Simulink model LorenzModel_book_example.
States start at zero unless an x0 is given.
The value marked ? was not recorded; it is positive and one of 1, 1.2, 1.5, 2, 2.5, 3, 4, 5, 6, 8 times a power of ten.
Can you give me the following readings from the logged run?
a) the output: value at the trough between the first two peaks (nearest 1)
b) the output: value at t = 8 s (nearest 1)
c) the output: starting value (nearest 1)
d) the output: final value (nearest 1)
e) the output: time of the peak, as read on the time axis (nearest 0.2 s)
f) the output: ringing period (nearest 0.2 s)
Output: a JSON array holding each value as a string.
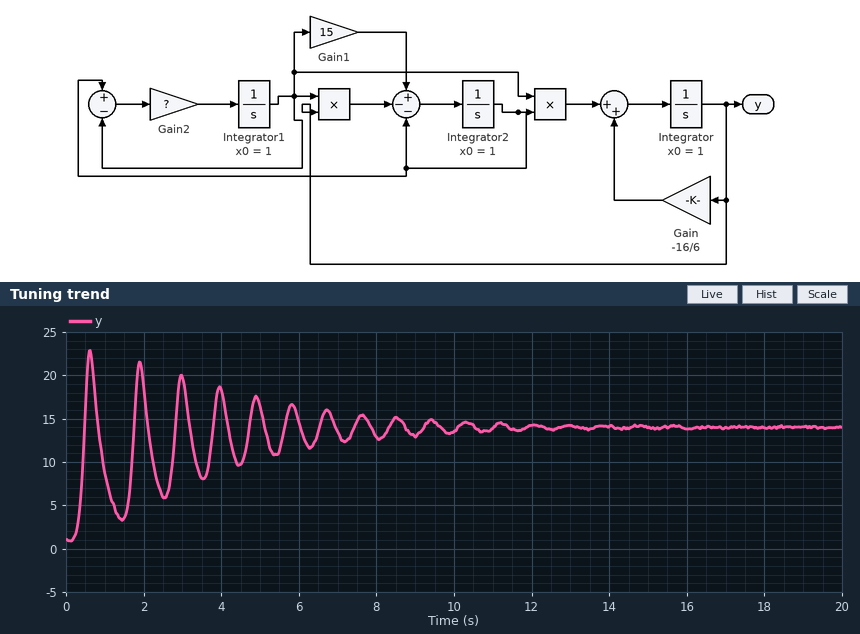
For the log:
["3", "13", "1", "14", "0.6 s", "1.2 s"]
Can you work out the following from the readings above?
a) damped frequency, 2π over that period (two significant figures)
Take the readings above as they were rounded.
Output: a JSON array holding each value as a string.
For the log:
["5.2 rad/s"]
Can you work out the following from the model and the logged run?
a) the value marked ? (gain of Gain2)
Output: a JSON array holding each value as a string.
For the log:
["6"]
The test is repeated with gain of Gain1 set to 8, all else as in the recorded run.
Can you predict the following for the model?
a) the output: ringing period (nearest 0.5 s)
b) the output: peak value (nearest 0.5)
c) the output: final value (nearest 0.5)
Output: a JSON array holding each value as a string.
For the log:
["1.5 s", "10.5", "7.0"]
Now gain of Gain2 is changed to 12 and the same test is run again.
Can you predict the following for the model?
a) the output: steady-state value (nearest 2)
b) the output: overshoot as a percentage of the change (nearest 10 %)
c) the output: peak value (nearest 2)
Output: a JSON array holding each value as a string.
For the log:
["14", "70 %", "24"]
